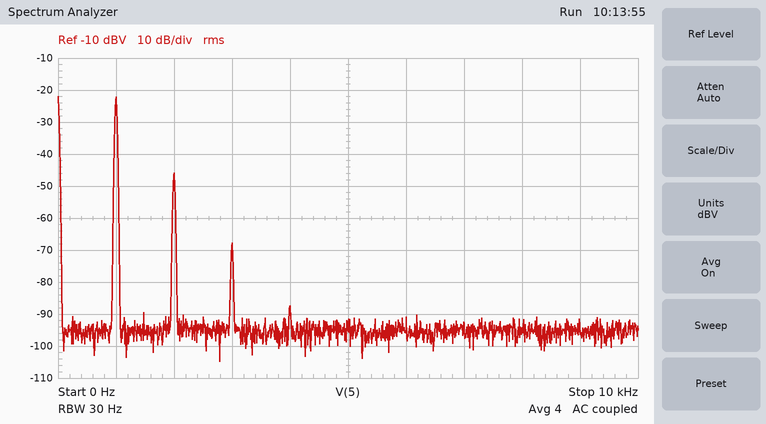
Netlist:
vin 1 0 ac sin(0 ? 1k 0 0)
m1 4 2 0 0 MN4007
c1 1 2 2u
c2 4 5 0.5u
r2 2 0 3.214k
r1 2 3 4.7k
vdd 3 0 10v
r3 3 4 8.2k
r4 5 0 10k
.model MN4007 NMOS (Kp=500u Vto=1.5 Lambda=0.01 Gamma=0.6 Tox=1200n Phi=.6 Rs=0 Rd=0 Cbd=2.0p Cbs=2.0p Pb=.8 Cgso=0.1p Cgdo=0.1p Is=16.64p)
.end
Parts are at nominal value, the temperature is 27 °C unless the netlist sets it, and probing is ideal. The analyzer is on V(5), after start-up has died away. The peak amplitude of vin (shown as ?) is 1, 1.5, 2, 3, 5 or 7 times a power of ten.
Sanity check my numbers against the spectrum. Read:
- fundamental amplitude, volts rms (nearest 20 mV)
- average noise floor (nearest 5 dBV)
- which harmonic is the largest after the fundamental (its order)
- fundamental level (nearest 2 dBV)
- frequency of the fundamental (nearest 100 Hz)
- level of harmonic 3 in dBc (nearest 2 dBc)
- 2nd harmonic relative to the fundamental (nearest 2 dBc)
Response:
80 mV
-95 dBV
2
-22 dBV
1.0 kHz
-46 dBc
-24 dBc
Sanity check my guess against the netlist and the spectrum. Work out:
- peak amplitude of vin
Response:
200 mV
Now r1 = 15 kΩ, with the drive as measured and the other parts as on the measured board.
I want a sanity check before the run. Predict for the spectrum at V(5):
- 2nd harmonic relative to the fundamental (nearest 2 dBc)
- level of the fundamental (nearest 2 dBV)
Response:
-14 dBc
-20 dBV
